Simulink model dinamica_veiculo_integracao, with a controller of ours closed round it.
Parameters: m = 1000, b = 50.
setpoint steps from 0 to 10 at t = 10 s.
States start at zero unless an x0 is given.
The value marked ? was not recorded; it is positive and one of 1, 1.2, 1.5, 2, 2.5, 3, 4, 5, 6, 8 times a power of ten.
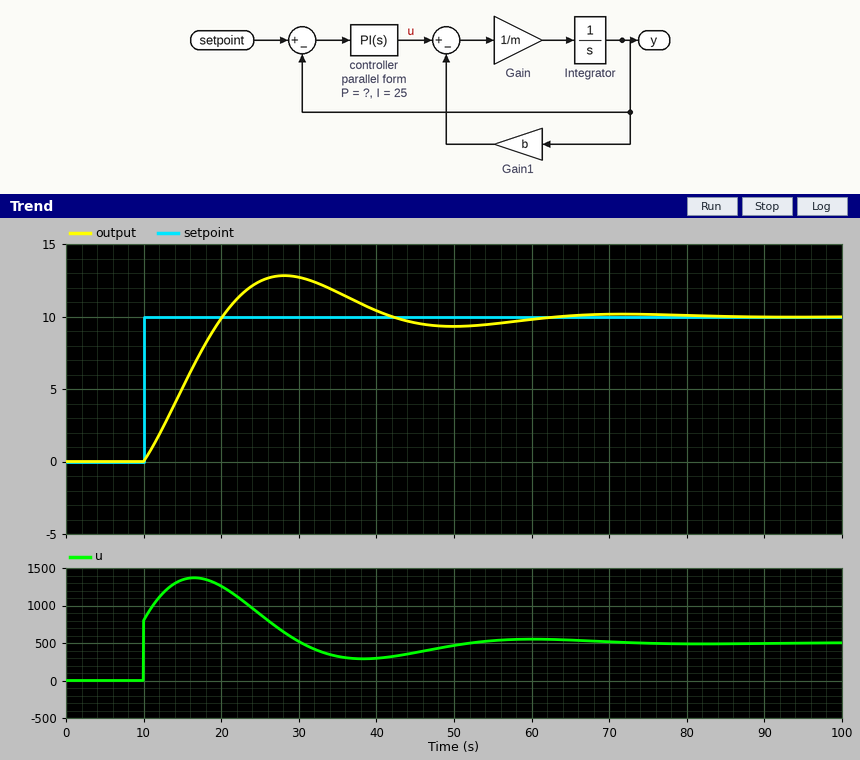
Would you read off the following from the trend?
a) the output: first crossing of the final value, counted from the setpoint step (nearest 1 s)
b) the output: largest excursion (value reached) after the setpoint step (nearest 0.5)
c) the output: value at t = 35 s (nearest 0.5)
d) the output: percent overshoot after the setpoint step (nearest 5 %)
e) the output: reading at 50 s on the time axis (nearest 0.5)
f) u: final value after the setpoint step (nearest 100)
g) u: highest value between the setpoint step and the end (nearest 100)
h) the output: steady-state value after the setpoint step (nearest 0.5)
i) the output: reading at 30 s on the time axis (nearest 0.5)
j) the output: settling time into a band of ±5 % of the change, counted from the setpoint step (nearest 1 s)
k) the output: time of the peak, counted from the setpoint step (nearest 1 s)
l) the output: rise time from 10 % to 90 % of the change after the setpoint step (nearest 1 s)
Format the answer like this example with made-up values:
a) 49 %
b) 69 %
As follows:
a) 10 s
b) 13.0
c) 11.5
d) 30 %
e) 9.5
f) 500
g) 1400
h) 10.0
i) 12.5
j) 45 s
k) 18 s
l) 8 s
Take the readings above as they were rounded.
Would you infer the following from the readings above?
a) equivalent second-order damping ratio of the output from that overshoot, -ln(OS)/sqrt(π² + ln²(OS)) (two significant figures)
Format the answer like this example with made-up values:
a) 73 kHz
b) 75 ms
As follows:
a) 0.36
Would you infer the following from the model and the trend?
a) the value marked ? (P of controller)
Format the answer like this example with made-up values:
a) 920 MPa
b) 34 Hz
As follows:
a) 80
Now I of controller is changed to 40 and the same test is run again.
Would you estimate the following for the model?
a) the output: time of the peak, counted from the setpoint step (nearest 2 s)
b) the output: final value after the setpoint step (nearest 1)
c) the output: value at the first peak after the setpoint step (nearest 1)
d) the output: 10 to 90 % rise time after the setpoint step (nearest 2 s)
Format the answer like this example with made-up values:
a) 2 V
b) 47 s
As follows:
a) 14 s
b) 10
c) 14
d) 6 s
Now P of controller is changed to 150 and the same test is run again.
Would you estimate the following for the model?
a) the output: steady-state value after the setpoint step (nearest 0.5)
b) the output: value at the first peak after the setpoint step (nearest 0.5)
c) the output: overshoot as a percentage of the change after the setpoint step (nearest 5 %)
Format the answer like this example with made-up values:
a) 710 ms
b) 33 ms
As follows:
a) 10.0
b) 11.5
c) 15 %
